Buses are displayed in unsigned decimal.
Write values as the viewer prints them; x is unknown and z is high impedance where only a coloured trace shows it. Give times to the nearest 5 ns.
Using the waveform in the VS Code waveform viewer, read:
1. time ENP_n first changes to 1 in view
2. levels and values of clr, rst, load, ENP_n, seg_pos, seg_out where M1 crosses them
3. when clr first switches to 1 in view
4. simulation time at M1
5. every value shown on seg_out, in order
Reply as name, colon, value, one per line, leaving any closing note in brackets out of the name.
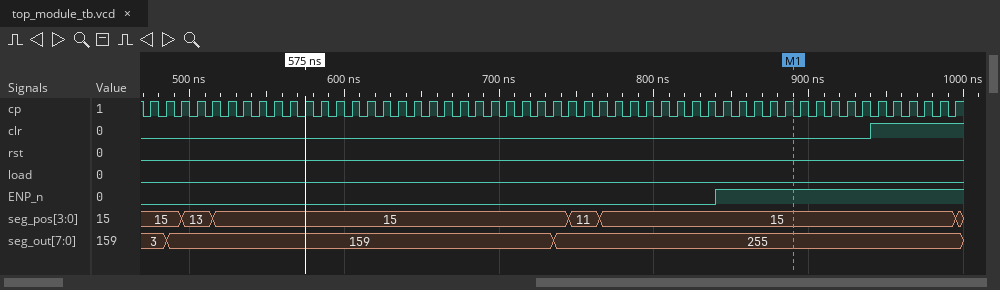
time ENP_n first changes to 1 in view: 840 ns
levels and values of clr, rst, load, ENP_n, seg_pos, seg_out where M1 crosses them: clr=0, rst=0, load=0, ENP_n=1, seg_pos=15, seg_out=255
when clr first switches to 1 in view: 940 ns
simulation time at M1: 890 ns
every value shown on seg_out, in order: 3, 159, 255
